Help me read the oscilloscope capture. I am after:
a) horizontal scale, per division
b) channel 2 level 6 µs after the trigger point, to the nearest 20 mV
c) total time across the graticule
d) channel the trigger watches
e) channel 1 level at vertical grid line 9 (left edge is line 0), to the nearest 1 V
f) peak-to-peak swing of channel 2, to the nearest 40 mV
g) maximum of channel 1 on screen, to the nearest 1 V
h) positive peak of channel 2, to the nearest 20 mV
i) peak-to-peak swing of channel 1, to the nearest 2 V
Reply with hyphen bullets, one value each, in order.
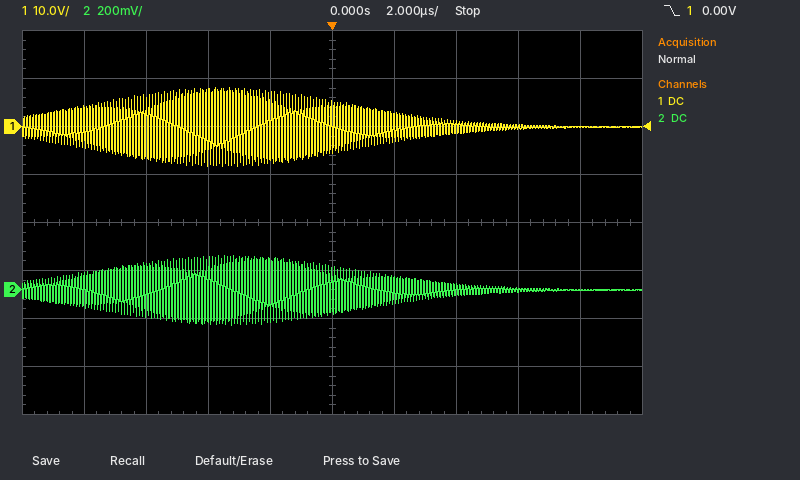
- 2 µs
- 0 mV
- 20 µs
- channel 1
- 0 V
- 280 mV
- 8 V
- 140 mV
- 16 V
